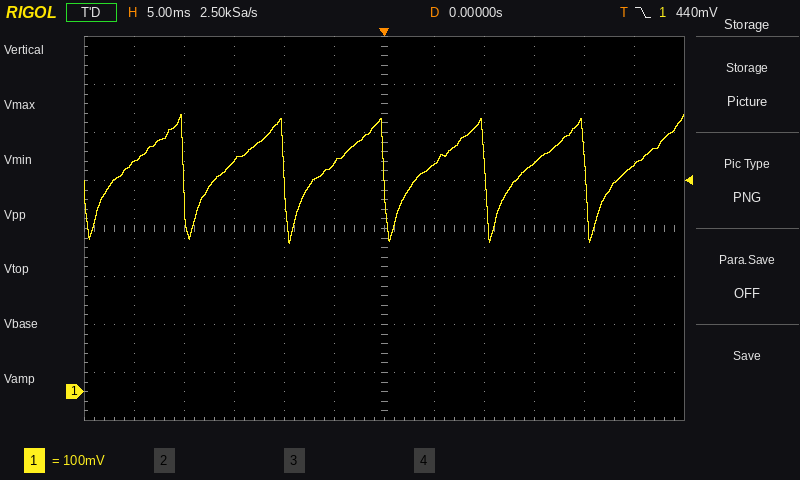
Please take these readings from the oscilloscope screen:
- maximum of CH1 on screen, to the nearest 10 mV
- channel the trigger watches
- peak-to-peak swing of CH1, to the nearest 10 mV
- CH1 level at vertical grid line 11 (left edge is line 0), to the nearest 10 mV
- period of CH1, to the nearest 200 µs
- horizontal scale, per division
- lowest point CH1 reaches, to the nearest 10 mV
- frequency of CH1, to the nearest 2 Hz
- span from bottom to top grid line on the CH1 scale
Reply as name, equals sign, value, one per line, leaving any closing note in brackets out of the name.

maximum of CH1 on screen, to the nearest 10 mV = 580 mV
channel the trigger watches = CH1
peak-to-peak swing of CH1, to the nearest 10 mV = 270 mV
CH1 level at vertical grid line 11 (left edge is line 0), to the nearest 10 mV = 470 mV
period of CH1, to the nearest 200 µs = 10.0 ms
horizontal scale, per division = 5 ms
lowest point CH1 reaches, to the nearest 10 mV = 310 mV
frequency of CH1, to the nearest 2 Hz = 100 Hz
span from bottom to top grid line on the CH1 scale = 800 mV
